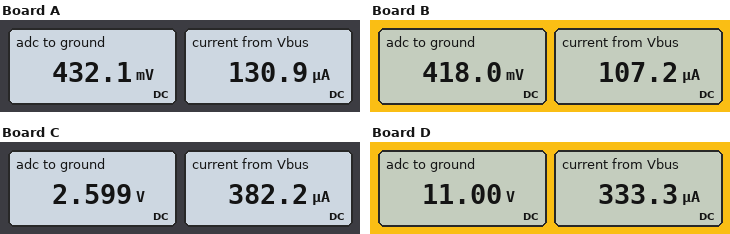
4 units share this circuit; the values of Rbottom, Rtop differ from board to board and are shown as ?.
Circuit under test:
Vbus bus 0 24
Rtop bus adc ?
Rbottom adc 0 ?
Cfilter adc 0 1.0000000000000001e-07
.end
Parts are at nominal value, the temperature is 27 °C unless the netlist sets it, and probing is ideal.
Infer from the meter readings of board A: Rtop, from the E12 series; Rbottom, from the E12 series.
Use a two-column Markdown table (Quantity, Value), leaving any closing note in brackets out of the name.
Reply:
| Quantity | Value |
|---|---|
| Rtop, from the E12 series | 180 kΩ |
| Rbottom, from the E12 series | 3.3 kΩ |
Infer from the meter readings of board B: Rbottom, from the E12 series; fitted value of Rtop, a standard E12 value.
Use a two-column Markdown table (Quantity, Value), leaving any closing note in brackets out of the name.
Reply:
| Quantity | Value |
|---|---|
| Rbottom, from the E12 series | 3.9 kΩ |
| fitted value of Rtop, a standard E12 value | 220 kΩ |
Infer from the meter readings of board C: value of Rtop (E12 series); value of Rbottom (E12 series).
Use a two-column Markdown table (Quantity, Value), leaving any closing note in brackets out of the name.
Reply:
| Quantity | Value |
|---|---|
| value of Rtop | 56 kΩ |
| value of Rbottom | 6.8 kΩ |
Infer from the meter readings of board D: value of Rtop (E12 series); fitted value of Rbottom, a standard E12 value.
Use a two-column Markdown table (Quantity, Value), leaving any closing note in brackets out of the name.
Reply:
| Quantity | Value |
|---|---|
| value of Rtop | 39 kΩ |
| fitted value of Rbottom, a standard E12 value | 33 kΩ |
